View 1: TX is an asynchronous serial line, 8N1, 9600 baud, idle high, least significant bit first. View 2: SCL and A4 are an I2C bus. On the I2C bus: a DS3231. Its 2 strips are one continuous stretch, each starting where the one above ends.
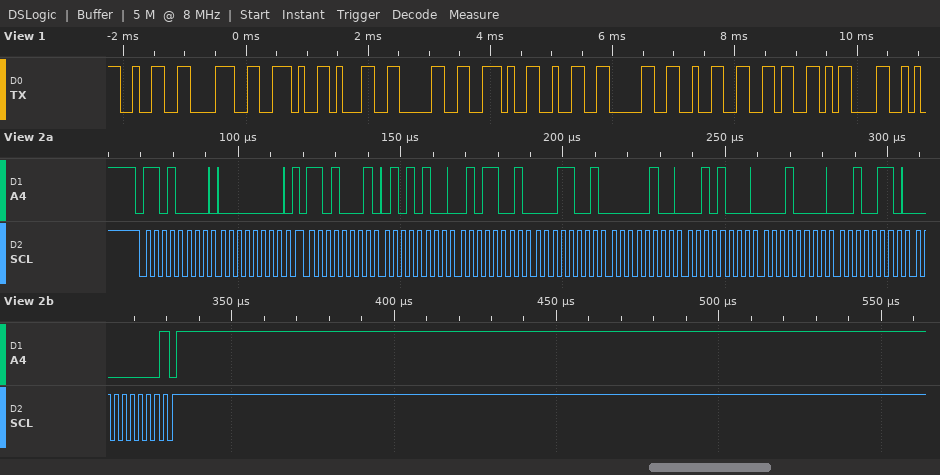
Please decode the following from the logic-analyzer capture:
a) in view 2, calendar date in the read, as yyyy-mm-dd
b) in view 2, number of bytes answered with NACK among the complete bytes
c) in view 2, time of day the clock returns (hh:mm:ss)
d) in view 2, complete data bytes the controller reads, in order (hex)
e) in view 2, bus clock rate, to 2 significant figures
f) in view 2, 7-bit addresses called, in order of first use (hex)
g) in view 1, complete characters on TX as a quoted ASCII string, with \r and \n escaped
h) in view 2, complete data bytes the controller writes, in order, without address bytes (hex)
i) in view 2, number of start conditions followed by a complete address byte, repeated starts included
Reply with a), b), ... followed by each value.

a) 2026-10-28
b) 1
c) 19:59:54
d) 54 59 19 04 28 10 26 00
e) 400 kHz
f) 0x68
g) "28.10.2026\r"
h) 00
i) 2
